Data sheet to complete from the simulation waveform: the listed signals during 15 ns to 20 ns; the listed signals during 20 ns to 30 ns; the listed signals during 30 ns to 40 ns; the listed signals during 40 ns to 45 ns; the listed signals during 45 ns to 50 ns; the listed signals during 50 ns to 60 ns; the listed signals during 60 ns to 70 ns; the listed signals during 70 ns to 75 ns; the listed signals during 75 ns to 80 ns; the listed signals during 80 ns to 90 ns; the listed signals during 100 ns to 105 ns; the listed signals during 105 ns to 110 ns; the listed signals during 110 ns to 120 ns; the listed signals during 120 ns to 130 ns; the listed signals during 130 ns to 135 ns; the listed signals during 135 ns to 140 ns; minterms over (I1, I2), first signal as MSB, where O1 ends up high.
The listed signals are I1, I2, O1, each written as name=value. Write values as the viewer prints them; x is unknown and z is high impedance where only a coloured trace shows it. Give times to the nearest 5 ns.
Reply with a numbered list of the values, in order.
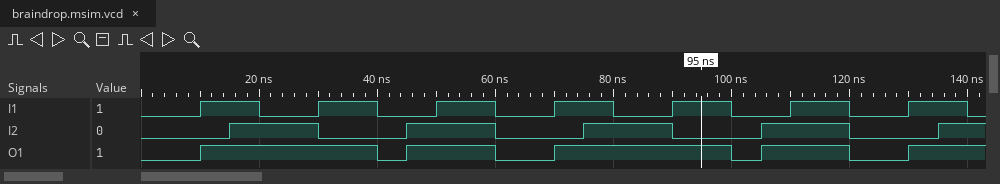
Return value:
1. I1=1, I2=1, O1=1
2. I1=0, I2=1, O1=1
3. I1=1, I2=0, O1=1
4. I1=0, I2=0, O1=0
5. I1=0, I2=1, O1=1
6. I1=1, I2=1, O1=1
7. I1=0, I2=0, O1=0
8. I1=1, I2=0, O1=1
9. I1=1, I2=1, O1=1
10. I1=0, I2=1, O1=1
11. I1=0, I2=0, O1=0
12. I1=0, I2=1, O1=1
13. I1=1, I2=1, O1=1
14. I1=0, I2=0, O1=0
15. I1=1, I2=0, O1=1
16. I1=1, I2=1, O1=1
17. 1, 2, 3
